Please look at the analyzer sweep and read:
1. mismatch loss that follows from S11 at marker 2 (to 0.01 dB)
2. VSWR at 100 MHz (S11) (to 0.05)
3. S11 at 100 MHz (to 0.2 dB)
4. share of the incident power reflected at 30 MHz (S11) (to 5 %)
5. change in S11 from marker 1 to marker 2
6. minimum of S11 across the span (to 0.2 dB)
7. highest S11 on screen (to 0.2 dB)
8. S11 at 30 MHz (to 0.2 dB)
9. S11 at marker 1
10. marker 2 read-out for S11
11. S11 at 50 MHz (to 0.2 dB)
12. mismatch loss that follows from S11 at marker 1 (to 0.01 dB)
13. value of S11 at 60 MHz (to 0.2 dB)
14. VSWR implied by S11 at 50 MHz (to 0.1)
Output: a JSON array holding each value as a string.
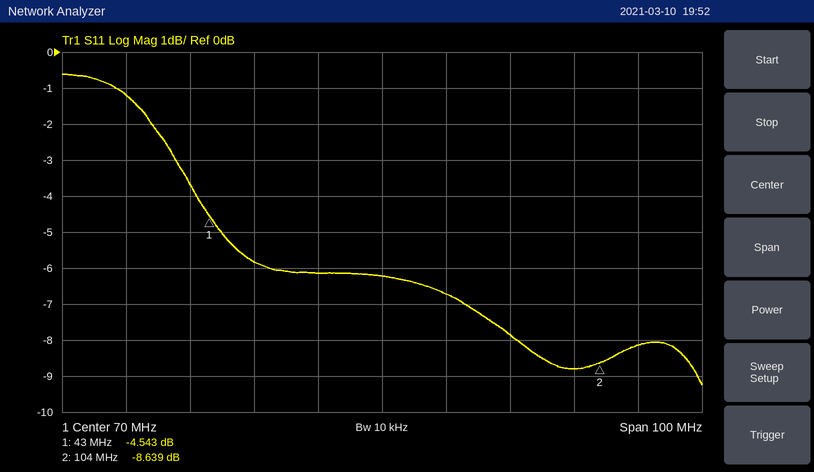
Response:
["0.64 dB", "2.15", "-8.8 dB", "75 %", "-4.096 dB", "-9.2 dB", "-0.6 dB", "-1.2 dB", "-4.543 dB", "-8.639 dB", "-5.8 dB", "1.88 dB", "-6.2 dB", "3.1"]
